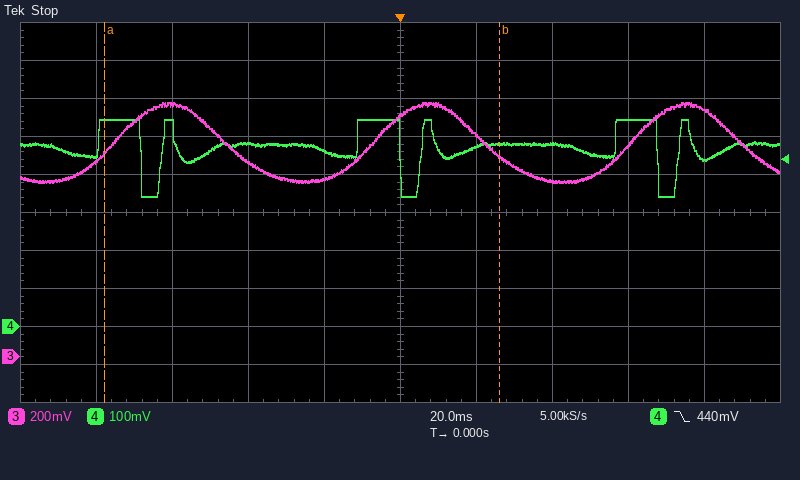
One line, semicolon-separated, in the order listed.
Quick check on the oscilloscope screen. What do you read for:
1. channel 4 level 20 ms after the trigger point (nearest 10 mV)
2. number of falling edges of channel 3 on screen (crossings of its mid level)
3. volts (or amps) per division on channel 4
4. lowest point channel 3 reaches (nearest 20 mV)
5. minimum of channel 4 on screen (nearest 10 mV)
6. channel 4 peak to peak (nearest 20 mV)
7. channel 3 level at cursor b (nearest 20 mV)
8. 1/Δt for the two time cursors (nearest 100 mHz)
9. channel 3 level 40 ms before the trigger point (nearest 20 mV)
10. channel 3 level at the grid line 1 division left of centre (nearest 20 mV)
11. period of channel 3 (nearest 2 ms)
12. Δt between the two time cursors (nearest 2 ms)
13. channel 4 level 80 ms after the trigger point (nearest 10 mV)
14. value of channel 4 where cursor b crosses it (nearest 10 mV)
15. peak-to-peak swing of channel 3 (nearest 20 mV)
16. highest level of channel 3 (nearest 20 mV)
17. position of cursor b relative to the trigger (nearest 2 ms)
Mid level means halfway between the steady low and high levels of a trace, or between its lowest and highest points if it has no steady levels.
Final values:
470 mV; 3; 100 mV; 920 mV; 340 mV; 200 mV; 1.06 V; 9.6 Hz; 1.02 V; 940 mV; 68 ms; 104 ms; 440 mV; 480 mV; 420 mV; 1.34 V; +26 ms
